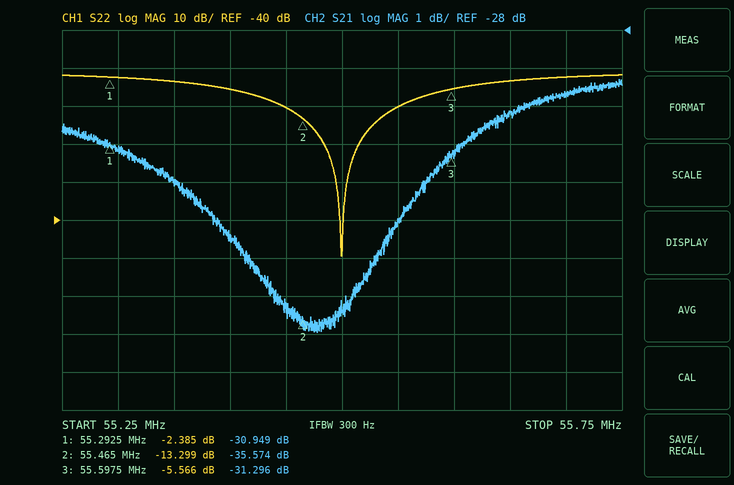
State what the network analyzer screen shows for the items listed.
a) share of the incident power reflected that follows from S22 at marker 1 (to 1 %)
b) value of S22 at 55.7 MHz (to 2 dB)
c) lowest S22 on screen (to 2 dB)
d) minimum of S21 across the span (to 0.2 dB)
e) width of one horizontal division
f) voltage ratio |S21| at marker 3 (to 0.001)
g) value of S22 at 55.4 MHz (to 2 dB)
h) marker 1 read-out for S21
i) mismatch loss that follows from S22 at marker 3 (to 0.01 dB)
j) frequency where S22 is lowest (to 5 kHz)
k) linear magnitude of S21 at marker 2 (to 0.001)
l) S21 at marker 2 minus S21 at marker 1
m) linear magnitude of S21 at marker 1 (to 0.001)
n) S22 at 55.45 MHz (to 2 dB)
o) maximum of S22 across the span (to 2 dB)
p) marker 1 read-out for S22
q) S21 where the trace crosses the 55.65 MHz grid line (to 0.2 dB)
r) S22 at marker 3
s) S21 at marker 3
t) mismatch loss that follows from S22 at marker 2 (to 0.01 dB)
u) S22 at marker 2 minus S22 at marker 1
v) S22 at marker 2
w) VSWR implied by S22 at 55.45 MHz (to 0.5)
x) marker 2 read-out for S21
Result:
58 %
-2 dB
-50 dB
-36.0 dB
50 kHz
0.027
-6 dB
-30.949 dB
1.41 dB
55.500 MHz
0.017
-4.625 dB
0.028
-10 dB
-2 dB
-2.385 dB
-30.2 dB
-5.566 dB
-31.296 dB
0.21 dB
-10.914 dB
-13.299 dB
2.0
-35.574 dB
